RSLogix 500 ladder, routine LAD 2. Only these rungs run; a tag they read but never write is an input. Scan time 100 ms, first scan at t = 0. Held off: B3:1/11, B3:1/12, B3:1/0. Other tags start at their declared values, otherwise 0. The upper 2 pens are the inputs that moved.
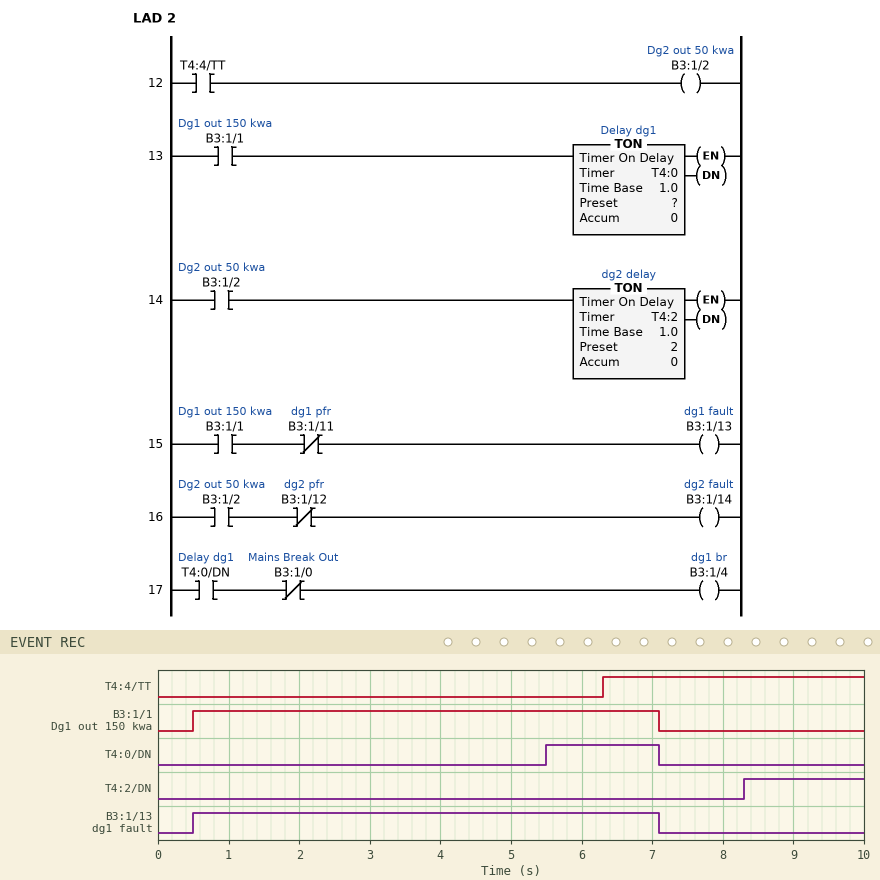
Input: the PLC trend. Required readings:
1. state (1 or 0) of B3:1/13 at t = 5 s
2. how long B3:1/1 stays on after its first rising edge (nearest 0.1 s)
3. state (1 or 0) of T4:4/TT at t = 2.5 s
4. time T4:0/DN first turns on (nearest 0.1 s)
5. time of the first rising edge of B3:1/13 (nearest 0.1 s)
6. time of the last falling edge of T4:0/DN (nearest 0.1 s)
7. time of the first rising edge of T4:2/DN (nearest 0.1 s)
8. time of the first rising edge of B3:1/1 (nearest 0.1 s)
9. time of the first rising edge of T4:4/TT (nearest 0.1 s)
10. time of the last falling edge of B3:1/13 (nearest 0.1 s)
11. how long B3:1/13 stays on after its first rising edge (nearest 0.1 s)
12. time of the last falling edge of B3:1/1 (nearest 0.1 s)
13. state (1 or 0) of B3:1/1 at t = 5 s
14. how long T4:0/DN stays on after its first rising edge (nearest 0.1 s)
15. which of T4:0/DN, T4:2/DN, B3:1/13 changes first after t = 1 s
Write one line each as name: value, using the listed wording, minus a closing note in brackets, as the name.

state (1 or 0) of B3:1/13 at t = 5 s: 1
how long B3:1/1 stays on after its first rising edge: 6.6 s
state (1 or 0) of T4:4/TT at t = 2.5 s: 0
time T4:0/DN first turns on: 5.5 s
time of the first rising edge of B3:1/13: 0.5 s
time of the last falling edge of T4:0/DN: 7.1 s
time of the first rising edge of T4:2/DN: 8.3 s
time of the first rising edge of B3:1/1: 0.5 s
time of the first rising edge of T4:4/TT: 6.3 s
time of the last falling edge of B3:1/13: 7.1 s
how long B3:1/13 stays on after its first rising edge: 6.6 s
time of the last falling edge of B3:1/1: 7.1 s
state (1 or 0) of B3:1/1 at t = 5 s: 1
how long T4:0/DN stays on after its first rising edge: 1.6 s
which of T4:0/DN, T4:2/DN, B3:1/13 changes first after t = 1 s: T4:0/DN
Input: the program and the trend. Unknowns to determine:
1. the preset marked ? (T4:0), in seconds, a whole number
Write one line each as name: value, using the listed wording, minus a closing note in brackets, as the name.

the preset marked ? (T4:0), in seconds, a whole number: 5 s
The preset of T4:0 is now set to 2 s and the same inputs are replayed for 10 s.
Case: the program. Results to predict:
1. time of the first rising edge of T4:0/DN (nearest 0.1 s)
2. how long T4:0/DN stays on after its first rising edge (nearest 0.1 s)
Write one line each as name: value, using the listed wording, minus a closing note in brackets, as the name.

time of the first rising edge of T4:0/DN: 2.5 s
how long T4:0/DN stays on after its first rising edge: 4.6 s
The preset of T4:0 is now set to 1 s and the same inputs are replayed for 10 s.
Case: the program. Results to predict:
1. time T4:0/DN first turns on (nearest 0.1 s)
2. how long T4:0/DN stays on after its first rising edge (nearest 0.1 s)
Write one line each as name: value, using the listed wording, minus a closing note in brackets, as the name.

time T4:0/DN first turns on: 1.5 s
how long T4:0/DN stays on after its first rising edge: 5.6 s
